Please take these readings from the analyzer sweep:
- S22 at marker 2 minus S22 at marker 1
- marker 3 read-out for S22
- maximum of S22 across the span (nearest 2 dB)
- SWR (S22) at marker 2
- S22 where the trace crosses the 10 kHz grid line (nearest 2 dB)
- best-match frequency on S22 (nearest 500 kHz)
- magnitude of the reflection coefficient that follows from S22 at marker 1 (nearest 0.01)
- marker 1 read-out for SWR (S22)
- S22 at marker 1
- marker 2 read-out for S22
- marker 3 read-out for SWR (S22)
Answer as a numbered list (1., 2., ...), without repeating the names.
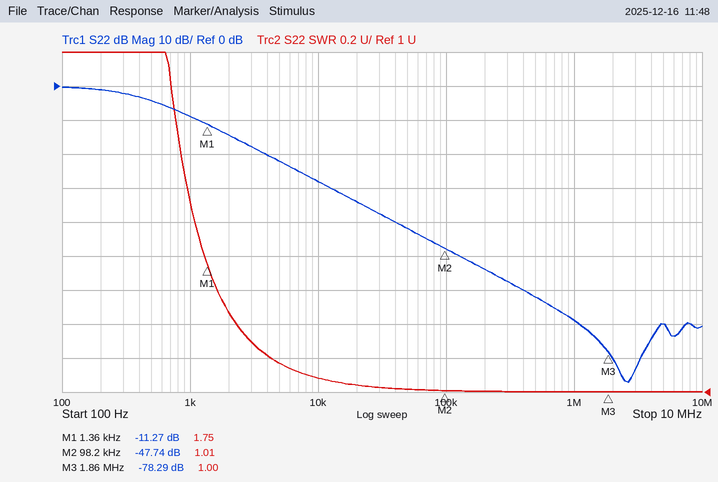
1. -36.47 dB
2. -78.29 dB
3. 0 dB
4. 1.01
5. -28 dB
6. 2.5 MHz
7. 0.27
8. 1.75
9. -11.27 dB
10. -47.74 dB
11. 1.00
